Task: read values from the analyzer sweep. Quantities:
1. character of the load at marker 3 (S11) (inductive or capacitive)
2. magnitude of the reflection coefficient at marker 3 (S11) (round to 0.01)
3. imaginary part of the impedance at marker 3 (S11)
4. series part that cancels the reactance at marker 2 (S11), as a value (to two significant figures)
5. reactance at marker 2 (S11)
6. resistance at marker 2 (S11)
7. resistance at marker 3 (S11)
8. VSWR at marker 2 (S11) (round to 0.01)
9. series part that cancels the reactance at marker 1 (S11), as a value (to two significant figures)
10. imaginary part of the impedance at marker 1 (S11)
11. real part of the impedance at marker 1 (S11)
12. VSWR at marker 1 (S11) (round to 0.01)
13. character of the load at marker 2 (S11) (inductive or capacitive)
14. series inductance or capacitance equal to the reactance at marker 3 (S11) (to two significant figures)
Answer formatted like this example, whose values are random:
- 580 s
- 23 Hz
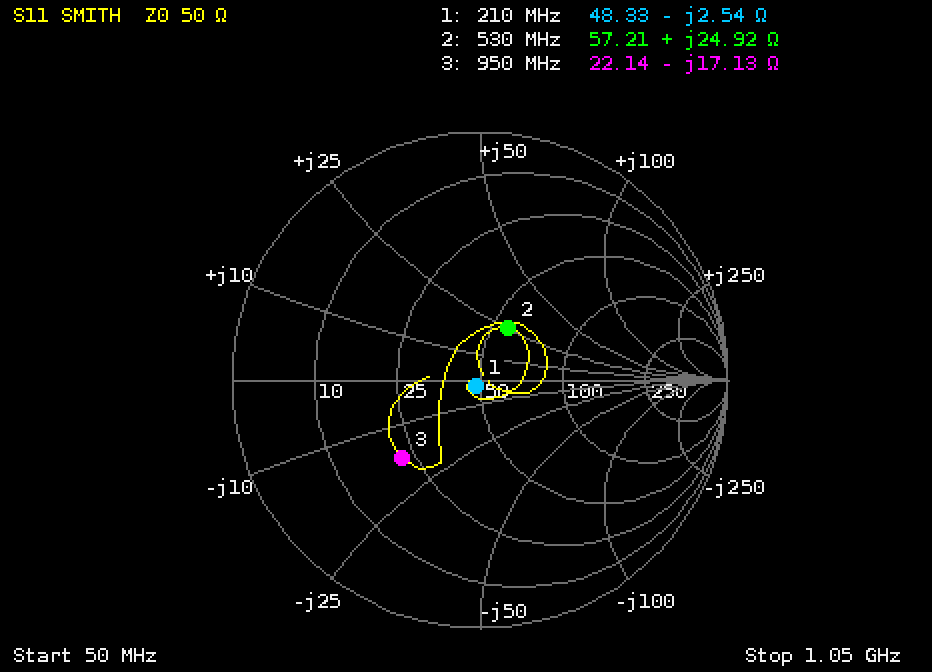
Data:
- capacitive
- 0.44
- -17.13 Ω
- 12 pF
- +24.92 Ω
- 57.21 Ω
- 22.14 Ω
- 1.62
- 1.9 nH
- -2.54 Ω
- 48.33 Ω
- 1.06
- inductive
- 9.8 pF
